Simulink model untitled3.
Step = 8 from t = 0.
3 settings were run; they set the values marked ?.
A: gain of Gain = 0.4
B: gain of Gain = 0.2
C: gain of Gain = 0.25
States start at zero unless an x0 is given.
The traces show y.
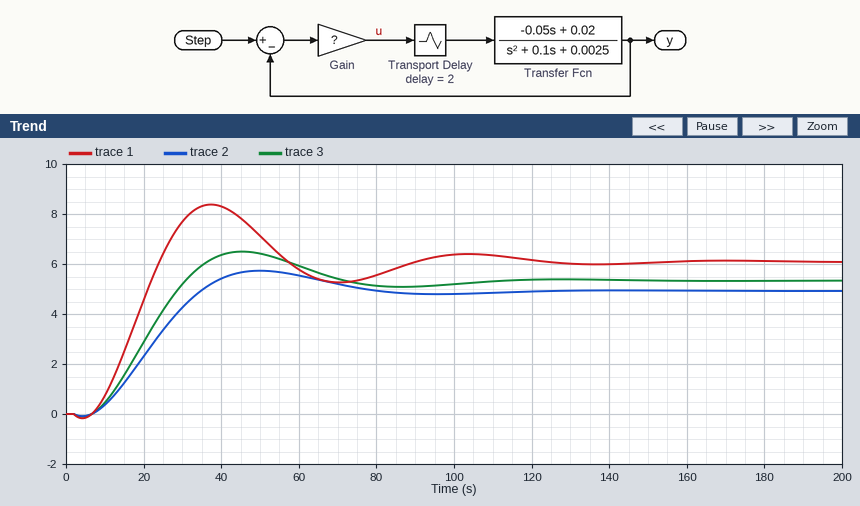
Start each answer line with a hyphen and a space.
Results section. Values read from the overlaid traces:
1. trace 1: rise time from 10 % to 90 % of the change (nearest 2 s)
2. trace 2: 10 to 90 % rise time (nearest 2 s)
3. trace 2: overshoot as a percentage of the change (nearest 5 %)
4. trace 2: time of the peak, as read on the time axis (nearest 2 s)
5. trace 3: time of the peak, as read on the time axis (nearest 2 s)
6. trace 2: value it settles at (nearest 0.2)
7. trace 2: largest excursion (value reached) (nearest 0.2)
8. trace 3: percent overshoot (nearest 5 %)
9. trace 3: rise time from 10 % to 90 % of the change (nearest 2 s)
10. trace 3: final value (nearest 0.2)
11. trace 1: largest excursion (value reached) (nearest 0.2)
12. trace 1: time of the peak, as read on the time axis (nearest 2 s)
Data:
- 12 s
- 20 s
- 15 %
- 50 s
- 46 s
- 5.0
- 5.8
- 20 %
- 18 s
- 5.4
- 8.4
- 38 s
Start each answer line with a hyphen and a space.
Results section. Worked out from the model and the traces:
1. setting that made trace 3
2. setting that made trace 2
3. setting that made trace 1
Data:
- C
- B
- A
